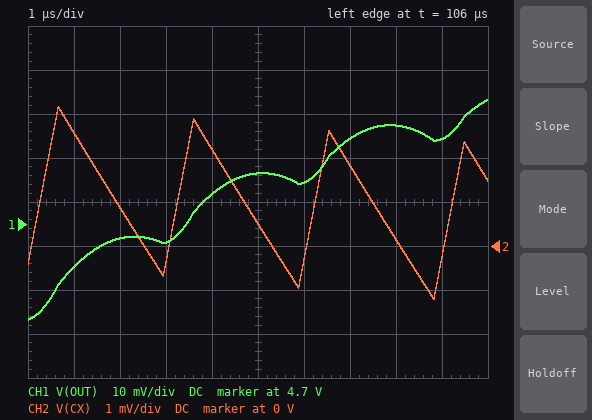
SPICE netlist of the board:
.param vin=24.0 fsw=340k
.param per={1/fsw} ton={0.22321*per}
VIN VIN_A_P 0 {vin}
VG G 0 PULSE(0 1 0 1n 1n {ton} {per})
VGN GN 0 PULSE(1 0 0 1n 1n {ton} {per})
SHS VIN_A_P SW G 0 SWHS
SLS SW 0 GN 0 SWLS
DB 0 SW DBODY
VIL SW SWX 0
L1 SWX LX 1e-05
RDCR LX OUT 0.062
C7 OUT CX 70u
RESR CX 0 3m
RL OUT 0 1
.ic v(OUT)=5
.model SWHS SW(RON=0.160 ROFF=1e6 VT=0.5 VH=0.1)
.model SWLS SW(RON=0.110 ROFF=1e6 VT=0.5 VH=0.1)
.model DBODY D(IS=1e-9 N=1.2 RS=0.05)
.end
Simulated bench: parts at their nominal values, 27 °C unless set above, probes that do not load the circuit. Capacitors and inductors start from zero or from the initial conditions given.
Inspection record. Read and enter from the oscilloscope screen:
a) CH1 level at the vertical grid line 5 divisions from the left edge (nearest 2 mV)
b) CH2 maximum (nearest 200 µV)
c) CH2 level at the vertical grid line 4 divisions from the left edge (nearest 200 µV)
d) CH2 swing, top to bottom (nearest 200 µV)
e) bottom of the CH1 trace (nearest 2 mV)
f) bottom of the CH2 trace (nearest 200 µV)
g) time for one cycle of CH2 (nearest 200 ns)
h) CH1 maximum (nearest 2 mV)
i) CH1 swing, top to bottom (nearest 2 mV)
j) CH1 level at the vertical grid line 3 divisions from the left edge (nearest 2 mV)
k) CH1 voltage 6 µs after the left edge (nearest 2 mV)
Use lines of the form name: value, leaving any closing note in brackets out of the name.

CH1 level at the vertical grid line 5 divisions from the left edge: 4.712 V
CH2 maximum: 3.2 mV
CH2 level at the vertical grid line 4 divisions from the left edge: 2.2 mV
CH2 swing, top to bottom: 4.4 mV
bottom of the CH1 trace: 4.678 V
bottom of the CH2 trace: -1.2 mV
time for one cycle of CH2: 3.0 µs
CH1 maximum: 4.728 V
CH1 swing, top to bottom: 50 mV
CH1 level at the vertical grid line 3 divisions from the left edge: 4.696 V
CH1 voltage 6 µs after the left edge: 4.710 V
